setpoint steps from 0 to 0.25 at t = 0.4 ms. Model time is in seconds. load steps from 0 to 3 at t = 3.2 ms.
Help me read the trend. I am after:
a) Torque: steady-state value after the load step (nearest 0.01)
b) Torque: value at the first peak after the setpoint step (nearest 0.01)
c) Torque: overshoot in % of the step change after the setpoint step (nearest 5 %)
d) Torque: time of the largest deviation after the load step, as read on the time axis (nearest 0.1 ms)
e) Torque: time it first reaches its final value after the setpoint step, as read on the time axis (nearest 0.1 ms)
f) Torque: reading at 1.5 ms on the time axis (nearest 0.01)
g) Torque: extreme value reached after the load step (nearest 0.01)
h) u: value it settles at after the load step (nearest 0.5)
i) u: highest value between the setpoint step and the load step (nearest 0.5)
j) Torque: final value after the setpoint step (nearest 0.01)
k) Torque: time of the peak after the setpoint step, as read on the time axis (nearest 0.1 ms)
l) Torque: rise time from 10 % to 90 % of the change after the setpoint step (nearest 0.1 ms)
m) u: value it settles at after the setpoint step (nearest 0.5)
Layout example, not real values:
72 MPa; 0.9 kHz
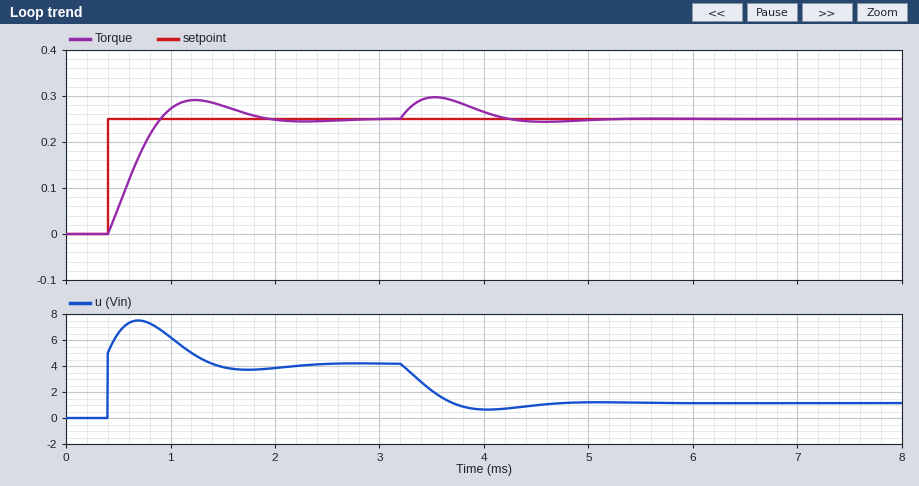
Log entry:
0.25; 0.29; 15 %; 3.5 ms; 0.9 ms; 0.28; 0.30; 1.0; 7.5; 0.25; 1.2 ms; 0.4 ms; 4.0
